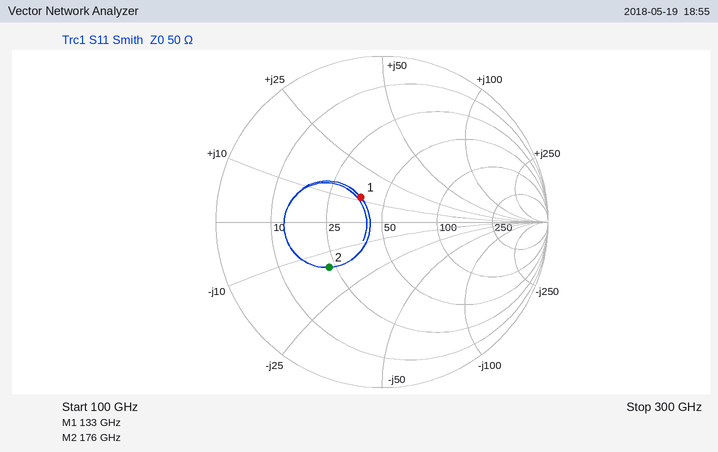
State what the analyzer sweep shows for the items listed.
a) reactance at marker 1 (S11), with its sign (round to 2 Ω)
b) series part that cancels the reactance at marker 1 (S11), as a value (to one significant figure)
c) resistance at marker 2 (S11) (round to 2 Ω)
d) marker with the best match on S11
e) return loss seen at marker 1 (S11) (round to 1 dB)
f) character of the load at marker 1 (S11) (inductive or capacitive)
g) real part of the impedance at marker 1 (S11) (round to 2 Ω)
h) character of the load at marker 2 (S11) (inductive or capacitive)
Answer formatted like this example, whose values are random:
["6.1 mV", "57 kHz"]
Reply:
["+12 Ω", "100 fF", "22 Ω", "marker 1", "14 dB", "inductive", "38 Ω", "capacitive"]
